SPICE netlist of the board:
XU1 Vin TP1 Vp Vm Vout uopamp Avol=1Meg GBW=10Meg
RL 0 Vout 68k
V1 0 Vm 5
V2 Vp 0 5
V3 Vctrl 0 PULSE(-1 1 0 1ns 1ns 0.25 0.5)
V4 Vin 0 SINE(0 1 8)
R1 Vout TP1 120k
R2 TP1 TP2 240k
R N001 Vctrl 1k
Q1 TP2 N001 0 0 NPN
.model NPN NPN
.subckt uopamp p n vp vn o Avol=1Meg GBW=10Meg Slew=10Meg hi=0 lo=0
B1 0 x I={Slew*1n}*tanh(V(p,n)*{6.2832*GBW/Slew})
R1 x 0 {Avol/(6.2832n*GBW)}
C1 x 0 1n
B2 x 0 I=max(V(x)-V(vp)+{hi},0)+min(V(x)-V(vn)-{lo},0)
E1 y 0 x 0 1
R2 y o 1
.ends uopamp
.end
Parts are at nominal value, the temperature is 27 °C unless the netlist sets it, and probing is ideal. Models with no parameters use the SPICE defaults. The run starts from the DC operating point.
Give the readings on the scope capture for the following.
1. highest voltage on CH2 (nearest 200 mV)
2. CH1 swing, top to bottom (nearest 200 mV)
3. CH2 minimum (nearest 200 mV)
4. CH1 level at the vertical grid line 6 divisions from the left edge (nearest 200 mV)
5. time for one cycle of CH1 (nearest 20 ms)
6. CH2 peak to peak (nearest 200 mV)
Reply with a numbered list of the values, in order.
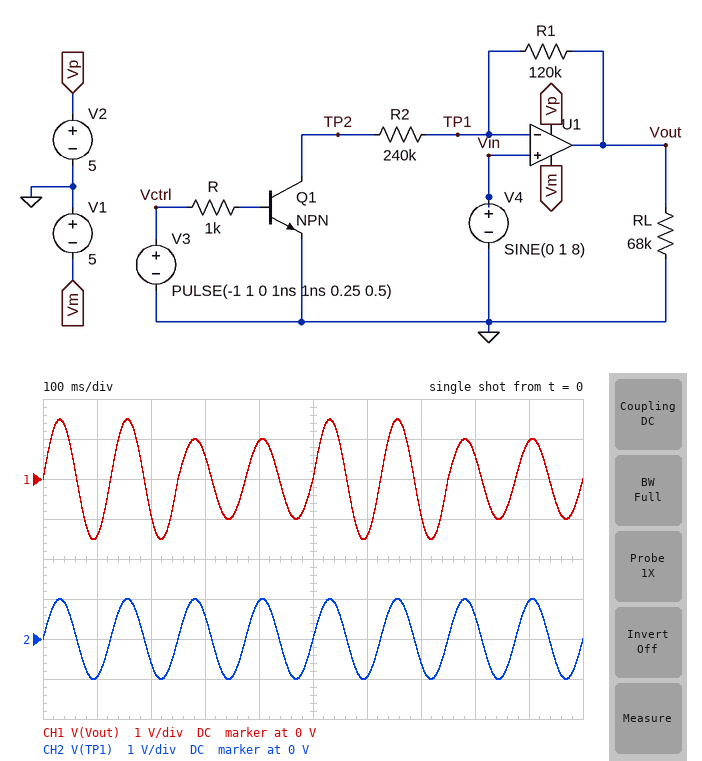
1. 1.0 V
2. 3.0 V
3. -1.0 V
4. -1.4 V
5. 120 ms
6. 2.0 V
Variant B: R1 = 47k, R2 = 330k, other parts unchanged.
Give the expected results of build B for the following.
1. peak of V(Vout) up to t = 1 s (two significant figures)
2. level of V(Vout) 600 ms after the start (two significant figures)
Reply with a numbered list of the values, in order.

1. 1.1 V
2. -1.1 V
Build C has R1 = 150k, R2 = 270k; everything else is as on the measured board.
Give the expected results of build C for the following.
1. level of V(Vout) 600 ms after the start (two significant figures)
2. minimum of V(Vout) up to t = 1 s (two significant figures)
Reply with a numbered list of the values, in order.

1. -1.5 V
2. -1.6 V
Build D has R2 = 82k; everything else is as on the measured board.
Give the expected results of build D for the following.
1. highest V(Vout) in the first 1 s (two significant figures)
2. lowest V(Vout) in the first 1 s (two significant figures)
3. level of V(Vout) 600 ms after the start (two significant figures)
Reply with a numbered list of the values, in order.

1. 2.4 V
2. -2.5 V
3. -2.4 V
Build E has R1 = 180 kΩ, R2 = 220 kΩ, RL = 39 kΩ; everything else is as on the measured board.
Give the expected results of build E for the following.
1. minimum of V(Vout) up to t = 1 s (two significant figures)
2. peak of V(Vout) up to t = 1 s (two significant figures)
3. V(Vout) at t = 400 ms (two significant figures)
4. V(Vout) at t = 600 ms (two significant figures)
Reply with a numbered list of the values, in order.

1. -1.8 V
2. 1.8 V
3. 950 mV
4. -1.7 V
